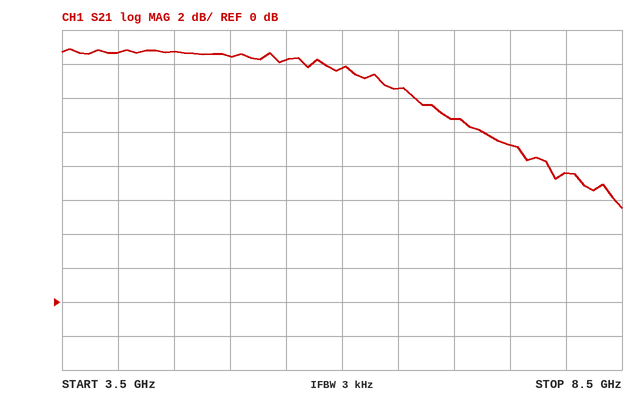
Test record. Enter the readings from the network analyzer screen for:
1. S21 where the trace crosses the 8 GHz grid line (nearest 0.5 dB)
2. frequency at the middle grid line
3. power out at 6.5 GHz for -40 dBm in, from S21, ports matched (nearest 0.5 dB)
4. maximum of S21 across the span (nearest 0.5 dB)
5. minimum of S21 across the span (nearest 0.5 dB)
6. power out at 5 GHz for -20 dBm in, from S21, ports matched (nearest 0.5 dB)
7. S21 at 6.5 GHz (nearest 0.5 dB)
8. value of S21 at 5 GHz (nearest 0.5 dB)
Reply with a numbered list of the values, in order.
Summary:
1. 7.5 dB
2. 6 GHz
3. -27.5 dBm
4. 15.0 dB
5. 5.5 dB
6. -5.5 dBm
7. 12.5 dB
8. 14.5 dB
